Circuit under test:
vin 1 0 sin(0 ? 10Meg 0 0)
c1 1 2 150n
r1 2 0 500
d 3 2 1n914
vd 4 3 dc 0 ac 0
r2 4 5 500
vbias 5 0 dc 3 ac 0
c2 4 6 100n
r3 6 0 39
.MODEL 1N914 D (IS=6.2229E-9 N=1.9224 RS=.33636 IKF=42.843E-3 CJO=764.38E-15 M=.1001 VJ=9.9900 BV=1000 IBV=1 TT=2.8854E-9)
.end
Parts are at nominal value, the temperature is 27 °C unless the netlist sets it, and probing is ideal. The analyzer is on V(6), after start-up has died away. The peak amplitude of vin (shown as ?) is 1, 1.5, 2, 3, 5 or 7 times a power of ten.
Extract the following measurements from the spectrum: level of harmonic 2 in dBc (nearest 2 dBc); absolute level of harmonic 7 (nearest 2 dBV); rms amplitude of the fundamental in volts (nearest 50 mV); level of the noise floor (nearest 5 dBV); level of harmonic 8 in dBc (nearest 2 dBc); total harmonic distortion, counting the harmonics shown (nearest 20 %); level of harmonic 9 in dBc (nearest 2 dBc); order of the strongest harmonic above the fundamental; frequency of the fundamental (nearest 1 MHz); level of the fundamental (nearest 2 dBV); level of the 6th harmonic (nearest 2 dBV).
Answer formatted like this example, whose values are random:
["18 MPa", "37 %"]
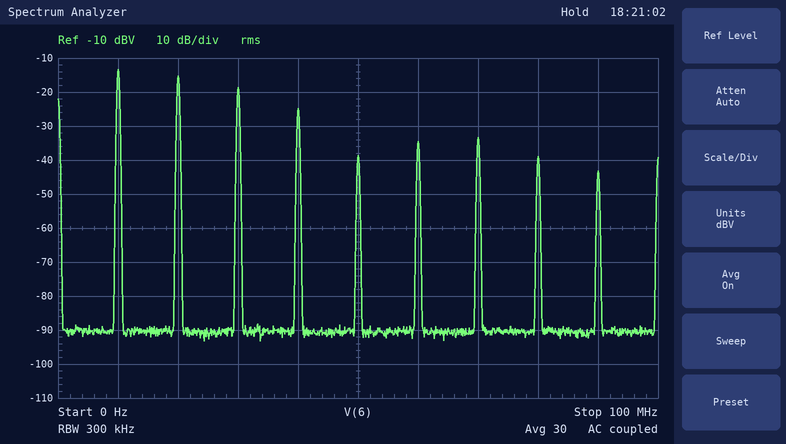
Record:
["-2 dBc", "-34 dBV", "200 mV", "-90 dBV", "-26 dBc", "100 %", "-30 dBc", "2", "10 MHz", "-14 dBV", "-34 dBV"]
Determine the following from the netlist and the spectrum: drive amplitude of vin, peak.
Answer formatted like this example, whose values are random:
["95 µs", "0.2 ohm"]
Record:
["3 V"]
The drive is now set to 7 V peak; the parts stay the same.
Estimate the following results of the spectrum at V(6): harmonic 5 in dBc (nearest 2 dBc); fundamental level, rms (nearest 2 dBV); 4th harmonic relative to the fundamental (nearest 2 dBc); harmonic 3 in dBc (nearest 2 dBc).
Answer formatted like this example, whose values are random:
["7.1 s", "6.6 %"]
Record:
["-16 dBc", "-8 dBV", "-8 dBc", "-4 dBc"]
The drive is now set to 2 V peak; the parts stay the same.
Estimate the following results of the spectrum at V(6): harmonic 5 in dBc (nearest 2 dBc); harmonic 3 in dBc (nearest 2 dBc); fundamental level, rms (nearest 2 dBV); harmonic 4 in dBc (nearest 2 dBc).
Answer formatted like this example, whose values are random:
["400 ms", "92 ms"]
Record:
["-28 dBc", "-6 dBc", "-16 dBV", "-14 dBc"]
